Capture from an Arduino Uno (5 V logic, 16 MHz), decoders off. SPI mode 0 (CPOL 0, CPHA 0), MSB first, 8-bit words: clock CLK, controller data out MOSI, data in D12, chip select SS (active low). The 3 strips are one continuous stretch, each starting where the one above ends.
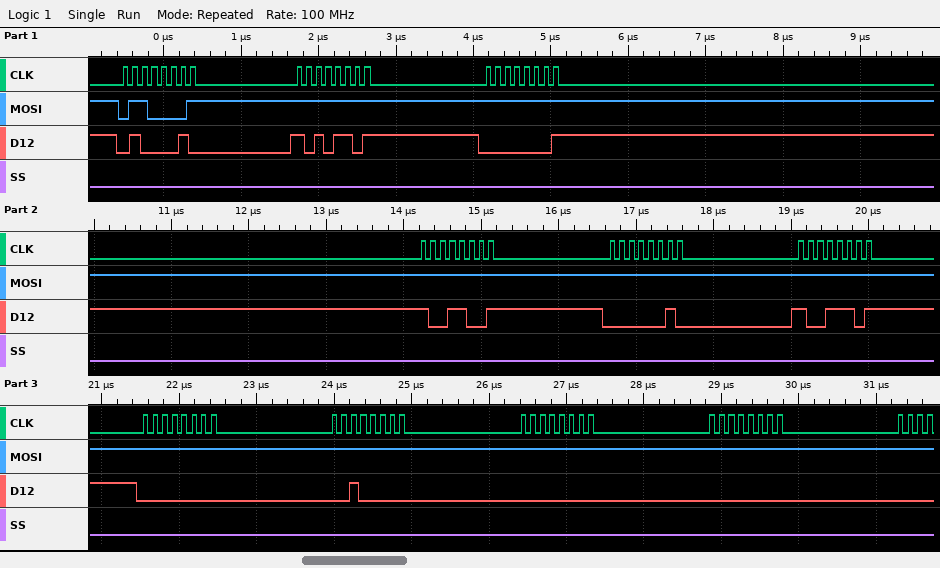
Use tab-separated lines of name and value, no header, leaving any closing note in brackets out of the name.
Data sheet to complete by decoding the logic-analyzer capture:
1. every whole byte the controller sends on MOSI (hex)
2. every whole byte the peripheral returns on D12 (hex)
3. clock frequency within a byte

every whole byte the controller sends on MOSI	61 FF FF FF FF FF FF FF FF FF
every whole byte the peripheral returns on D12	42 AD 01 99 02 9D 00 20 00 00
clock frequency within a byte	8 MHz
